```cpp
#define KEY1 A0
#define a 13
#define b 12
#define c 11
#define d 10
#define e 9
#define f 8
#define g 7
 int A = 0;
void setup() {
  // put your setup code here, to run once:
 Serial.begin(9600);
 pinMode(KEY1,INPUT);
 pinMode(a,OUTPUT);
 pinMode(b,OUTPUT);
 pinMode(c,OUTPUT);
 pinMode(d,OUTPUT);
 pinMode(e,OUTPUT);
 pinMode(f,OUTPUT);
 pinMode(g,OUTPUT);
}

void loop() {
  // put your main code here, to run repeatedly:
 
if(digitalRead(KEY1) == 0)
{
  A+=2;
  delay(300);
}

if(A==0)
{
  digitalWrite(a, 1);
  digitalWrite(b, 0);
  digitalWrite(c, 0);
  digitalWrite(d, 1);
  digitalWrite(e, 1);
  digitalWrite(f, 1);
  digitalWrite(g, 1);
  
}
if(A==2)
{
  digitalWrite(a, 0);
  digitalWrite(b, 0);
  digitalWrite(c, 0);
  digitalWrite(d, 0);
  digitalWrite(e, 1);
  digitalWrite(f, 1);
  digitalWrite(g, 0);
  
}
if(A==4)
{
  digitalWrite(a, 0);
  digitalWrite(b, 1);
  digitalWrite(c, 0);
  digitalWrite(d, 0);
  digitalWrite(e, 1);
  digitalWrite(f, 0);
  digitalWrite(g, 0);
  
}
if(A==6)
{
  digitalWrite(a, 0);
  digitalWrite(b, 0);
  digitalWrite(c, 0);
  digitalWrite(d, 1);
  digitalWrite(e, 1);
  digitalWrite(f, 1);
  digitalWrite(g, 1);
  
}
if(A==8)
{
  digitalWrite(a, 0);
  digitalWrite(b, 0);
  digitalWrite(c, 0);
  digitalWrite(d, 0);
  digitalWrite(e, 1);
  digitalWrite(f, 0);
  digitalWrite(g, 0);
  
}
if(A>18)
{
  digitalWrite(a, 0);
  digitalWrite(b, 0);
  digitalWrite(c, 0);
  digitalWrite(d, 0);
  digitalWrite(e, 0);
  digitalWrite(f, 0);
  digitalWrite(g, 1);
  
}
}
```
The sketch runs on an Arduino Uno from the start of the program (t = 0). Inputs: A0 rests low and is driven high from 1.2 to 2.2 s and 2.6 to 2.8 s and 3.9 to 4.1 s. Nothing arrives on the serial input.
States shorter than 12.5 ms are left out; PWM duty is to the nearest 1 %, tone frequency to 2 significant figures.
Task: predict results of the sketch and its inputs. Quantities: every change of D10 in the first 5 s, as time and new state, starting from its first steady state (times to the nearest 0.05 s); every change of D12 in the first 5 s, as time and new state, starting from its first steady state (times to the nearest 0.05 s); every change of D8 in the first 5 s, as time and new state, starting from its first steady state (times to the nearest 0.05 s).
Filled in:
0 s low; 0.9 s high; 1.2 s low
0 s low; 0.6 s high; 0.9 s low
0 s low; 0.3 s high; 0.6 s low; 0.9 s high; 1.2 s low
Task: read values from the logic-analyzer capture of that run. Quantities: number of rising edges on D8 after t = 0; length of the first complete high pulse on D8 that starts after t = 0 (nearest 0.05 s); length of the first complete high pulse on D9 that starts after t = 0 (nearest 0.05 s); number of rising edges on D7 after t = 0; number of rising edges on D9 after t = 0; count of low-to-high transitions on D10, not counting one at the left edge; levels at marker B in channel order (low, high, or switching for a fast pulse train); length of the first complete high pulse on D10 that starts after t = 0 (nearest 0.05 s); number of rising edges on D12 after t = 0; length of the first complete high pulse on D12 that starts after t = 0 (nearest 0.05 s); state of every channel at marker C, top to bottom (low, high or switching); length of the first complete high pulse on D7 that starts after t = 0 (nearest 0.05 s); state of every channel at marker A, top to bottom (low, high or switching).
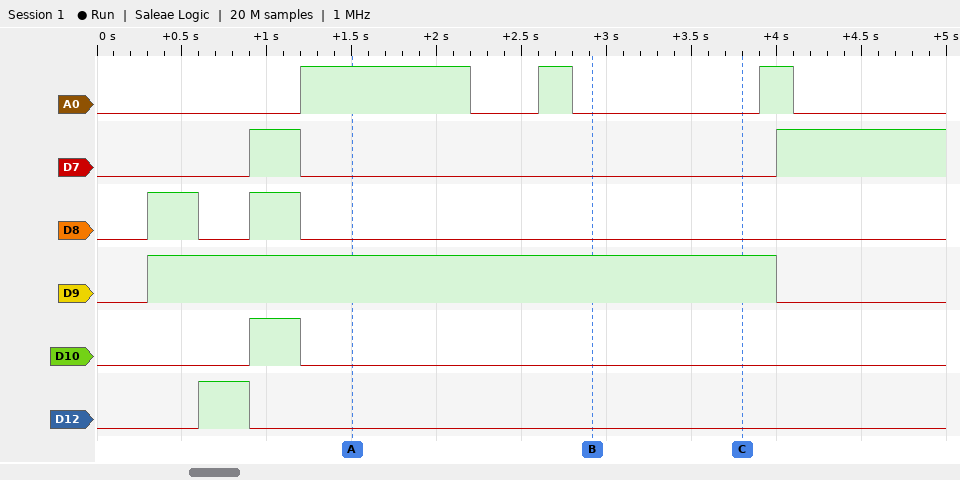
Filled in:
2
0.30 s
3.70 s
2
1
1
A0 low, D7 low, D8 low, D9 high, D10 low, D12 low
0.30 s
1
0.30 s
A0 low, D7 low, D8 low, D9 high, D10 low, D12 low
0.30 s
A0 high, D7 low, D8 low, D9 high, D10 low, D12 low
